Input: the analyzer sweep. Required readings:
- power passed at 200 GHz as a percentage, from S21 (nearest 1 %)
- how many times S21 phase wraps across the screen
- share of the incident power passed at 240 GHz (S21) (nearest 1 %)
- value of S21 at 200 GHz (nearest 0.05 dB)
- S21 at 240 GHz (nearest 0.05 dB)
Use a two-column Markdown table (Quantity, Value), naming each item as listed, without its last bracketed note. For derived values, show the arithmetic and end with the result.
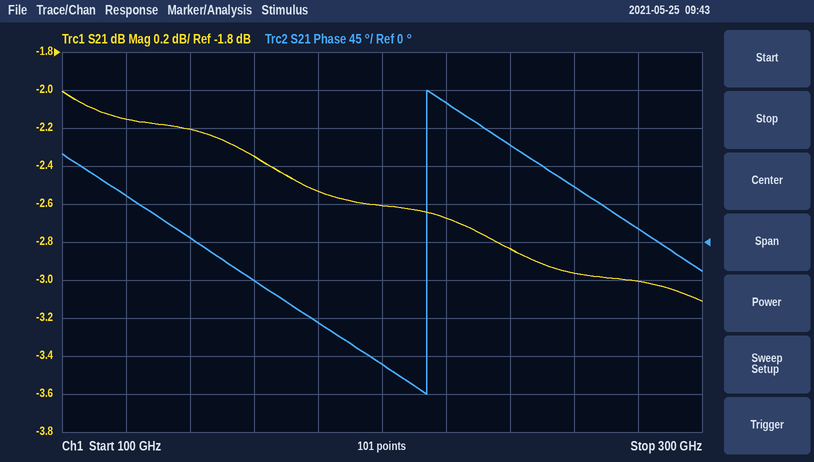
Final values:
| Quantity | Value |
|---|---|
| power passed at 200 GHz as a percentage, from S21 | 10^(-2.6/10) ≈ 55 % |
| how many times S21 phase wraps across the screen | 1 |
| share of the incident power passed at 240 GHz (S21) | 10^(-2.85/10) ≈ 52 % |
| value of S21 at 200 GHz | -2.60 dB |
| S21 at 240 GHz | -2.85 dB |
